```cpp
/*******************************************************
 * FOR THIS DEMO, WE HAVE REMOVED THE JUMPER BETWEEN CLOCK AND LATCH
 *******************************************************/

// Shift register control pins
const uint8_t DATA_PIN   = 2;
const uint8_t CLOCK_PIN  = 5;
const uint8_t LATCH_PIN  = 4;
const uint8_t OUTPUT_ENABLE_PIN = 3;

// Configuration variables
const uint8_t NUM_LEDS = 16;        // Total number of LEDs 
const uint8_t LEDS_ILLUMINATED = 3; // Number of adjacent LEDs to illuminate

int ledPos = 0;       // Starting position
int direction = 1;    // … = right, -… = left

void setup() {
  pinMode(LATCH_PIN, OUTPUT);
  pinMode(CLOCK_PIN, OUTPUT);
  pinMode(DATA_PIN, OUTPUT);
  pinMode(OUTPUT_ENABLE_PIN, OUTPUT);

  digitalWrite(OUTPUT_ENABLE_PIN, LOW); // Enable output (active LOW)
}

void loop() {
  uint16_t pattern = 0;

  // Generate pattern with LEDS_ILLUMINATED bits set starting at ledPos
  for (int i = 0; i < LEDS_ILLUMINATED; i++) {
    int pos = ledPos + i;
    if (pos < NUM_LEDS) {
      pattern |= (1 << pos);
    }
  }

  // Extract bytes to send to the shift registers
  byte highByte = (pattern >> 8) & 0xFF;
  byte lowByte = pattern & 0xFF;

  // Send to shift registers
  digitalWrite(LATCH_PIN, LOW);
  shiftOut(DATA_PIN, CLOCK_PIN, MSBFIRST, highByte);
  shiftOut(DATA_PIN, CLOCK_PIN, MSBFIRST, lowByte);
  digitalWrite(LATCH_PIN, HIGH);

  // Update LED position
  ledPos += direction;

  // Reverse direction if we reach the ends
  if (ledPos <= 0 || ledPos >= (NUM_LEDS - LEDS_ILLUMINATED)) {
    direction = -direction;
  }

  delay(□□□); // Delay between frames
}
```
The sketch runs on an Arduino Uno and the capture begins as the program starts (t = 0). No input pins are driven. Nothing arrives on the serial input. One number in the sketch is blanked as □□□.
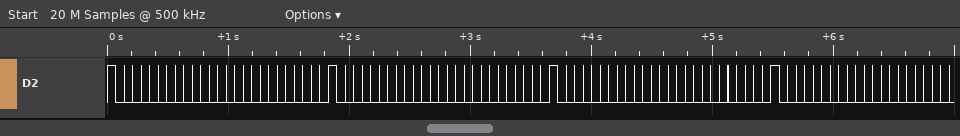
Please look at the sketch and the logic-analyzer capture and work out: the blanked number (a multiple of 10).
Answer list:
70
